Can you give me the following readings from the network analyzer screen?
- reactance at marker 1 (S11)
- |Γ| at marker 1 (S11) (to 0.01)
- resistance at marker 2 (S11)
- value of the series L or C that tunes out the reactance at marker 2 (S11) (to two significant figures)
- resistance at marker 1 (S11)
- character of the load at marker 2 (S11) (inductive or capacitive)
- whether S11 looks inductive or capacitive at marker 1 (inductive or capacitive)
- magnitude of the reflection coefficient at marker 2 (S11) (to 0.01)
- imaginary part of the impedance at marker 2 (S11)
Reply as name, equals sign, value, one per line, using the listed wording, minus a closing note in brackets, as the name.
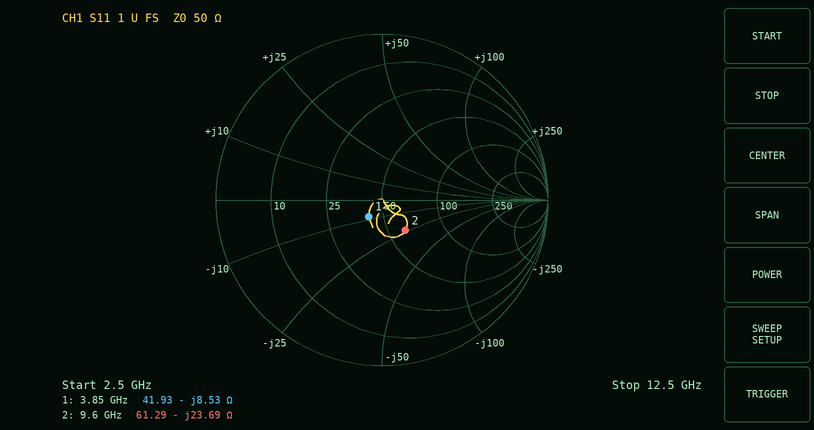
reactance at marker 1 = -8.53 Ω
|Γ| at marker 1 (S11) = 0.13
resistance at marker 2 = 61.29 Ω
value of the series L or C that tunes out the reactance at marker 2 (S11) = 390 pH
resistance at marker 1 = 41.93 Ω
character of the load at marker 2 (S11) = capacitive
whether S11 looks inductive or capacitive at marker 1 = capacitive
magnitude of the reflection coefficient at marker 2 (S11) = 0.23
imaginary part of the impedance at marker 2 = -23.69 Ω
